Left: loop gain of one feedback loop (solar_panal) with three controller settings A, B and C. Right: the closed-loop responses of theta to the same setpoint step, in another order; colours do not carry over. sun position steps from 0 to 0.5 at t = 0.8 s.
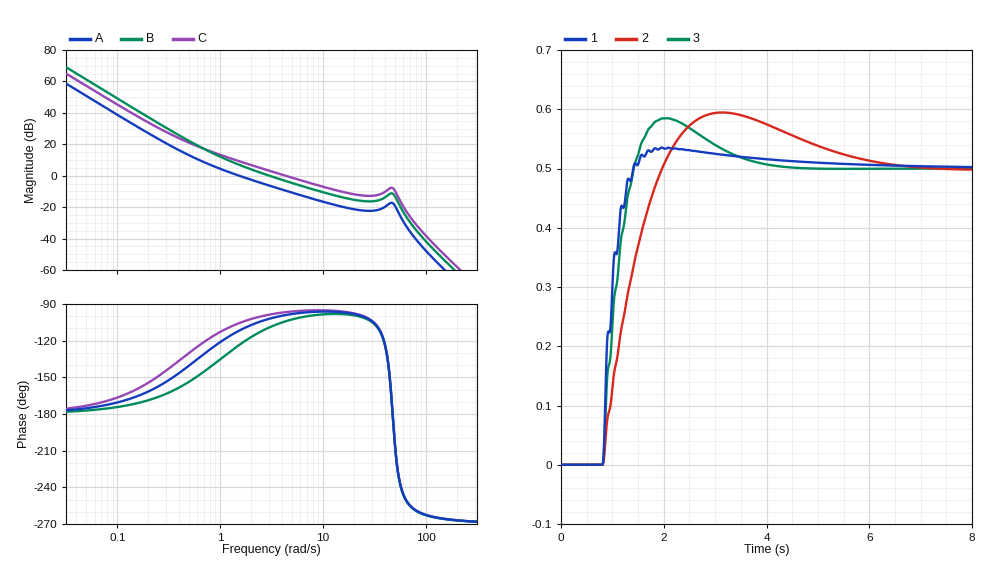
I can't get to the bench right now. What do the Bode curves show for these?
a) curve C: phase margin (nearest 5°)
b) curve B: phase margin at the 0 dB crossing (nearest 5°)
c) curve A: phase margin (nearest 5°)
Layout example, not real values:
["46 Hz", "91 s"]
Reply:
["85°", "70°", "70°"]
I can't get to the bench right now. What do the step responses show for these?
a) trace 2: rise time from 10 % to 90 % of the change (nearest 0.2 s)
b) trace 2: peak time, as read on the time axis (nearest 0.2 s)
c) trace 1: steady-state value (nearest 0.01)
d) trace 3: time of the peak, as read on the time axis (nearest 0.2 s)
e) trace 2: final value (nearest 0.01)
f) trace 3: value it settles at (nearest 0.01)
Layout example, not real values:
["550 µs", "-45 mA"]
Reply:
["0.8 s", "3.2 s", "0.50", "2.0 s", "0.50", "0.50"]
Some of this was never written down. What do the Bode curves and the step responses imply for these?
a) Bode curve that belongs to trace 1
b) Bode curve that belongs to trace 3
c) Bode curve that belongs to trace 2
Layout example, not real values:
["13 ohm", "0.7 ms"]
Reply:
["C", "B", "A"]
